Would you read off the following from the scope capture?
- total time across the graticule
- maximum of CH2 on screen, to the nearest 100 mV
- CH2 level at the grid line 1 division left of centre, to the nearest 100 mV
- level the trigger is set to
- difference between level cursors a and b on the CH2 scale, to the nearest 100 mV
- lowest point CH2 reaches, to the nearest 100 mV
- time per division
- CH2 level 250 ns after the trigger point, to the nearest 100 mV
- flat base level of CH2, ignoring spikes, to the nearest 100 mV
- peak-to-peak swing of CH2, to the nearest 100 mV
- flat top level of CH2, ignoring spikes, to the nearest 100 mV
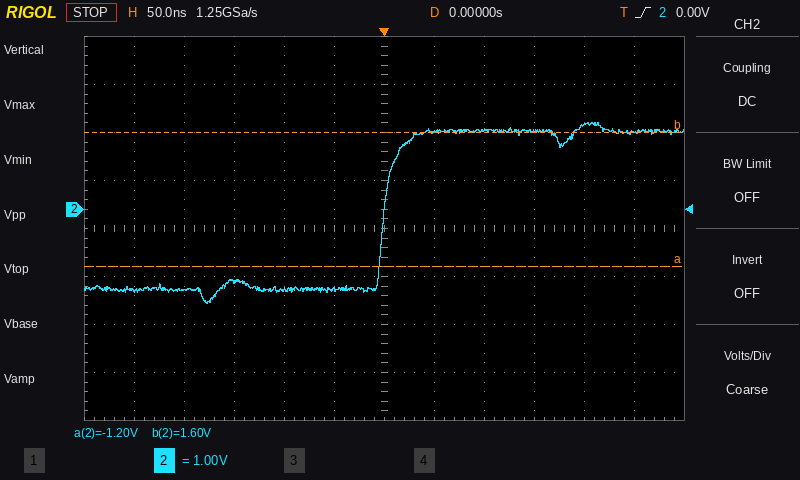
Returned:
600 ns
1.8 V
-1.7 V
0.00 V
2.8 V
-2.0 V
50 ns
1.6 V
-1.7 V
3.8 V
1.6 V
